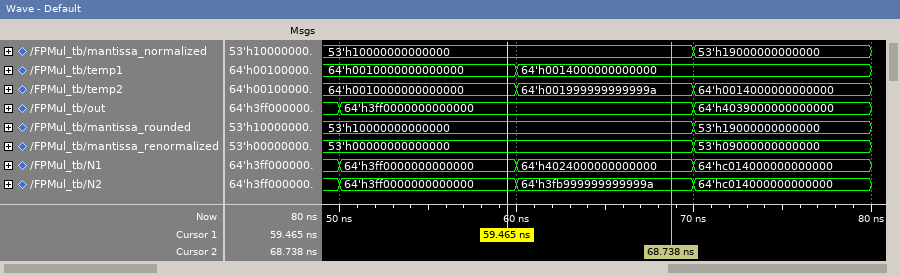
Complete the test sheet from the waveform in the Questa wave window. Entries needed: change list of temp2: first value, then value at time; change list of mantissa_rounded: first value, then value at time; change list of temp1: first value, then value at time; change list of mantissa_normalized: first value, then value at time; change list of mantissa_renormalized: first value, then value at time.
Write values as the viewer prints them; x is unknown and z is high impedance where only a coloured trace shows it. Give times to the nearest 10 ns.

64'h0010000000000000, 64'h001999999999999a at 60 ns, 64'h0014000000000000 at 70 ns
53'h10000000000000, 53'h19000000000000 at 70 ns
64'h0010000000000000, 64'h0014000000000000 at 60 ns
53'h10000000000000, 53'h19000000000000 at 70 ns
53'h00000000000000, 53'h09000000000000 at 70 ns
